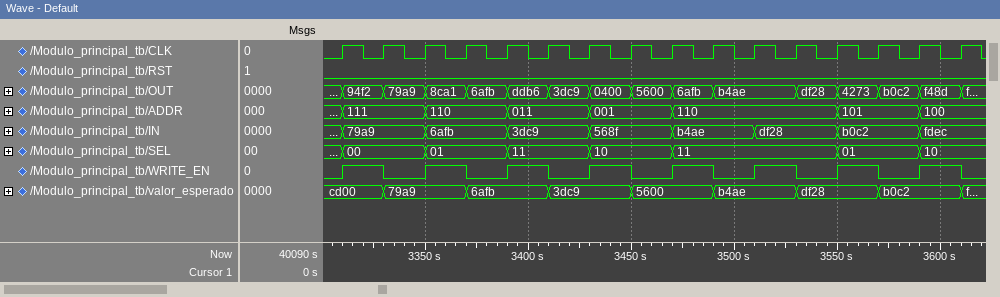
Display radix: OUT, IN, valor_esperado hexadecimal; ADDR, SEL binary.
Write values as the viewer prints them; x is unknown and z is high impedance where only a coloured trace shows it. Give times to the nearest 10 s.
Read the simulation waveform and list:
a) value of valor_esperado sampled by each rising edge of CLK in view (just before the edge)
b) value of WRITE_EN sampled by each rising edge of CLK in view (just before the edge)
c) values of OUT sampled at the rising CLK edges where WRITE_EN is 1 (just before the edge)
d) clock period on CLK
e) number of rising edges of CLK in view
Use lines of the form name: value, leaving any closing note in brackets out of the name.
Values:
value of valor_esperado sampled by each rising edge of CLK in view: cd00, cd00, 79a9, 79a9, 6afb, 6afb, 3dc9, 3dc9, 5600, 5600, b4ae, b4ae, df28, df28, b0c2, b0c2
value of WRITE_EN sampled by each rising edge of CLK in view: 0 1 0 1 0 1 0 1 0 1 0 1 0 1 0 1
values of OUT sampled at the rising CLK edges where WRITE_EN is 1: 94f2, 8ca1, ddb6, 0400, 6afb, b4ae, 4273, f48d
clock period on CLK: 20 s
number of rising edges of CLK in view: 16
